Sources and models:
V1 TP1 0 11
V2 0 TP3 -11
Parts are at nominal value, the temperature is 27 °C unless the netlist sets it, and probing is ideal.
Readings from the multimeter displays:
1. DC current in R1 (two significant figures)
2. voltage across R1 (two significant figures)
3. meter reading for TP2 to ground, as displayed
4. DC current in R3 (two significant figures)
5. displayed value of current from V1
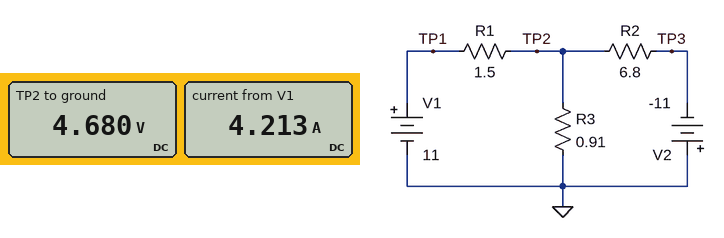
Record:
4.2 A
6.3 V
4.680 V
5.1 A
4.213 A
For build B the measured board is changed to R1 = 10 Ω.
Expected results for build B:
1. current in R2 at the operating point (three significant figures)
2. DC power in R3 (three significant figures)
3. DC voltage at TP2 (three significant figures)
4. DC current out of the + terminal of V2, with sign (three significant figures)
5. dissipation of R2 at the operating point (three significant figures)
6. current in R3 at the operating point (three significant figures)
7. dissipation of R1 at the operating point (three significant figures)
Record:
1.32 A
4.48 W
2.02 V
-1.32 A
11.9 W
2.22 A
8.07 W
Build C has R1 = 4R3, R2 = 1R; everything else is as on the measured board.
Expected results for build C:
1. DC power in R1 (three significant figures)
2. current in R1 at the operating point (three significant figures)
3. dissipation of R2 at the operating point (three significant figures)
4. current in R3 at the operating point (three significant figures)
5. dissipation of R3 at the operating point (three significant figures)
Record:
6.25 W
1.21 A
26.9 W
6.39 A
37.2 W
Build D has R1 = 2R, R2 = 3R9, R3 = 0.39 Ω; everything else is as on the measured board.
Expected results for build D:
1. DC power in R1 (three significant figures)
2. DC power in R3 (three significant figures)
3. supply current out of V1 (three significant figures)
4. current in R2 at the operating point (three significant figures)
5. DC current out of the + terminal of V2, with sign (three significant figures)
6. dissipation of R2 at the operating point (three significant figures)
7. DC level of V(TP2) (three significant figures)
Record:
36.1 W
16.1 W
4.25 A
2.18 A
-2.18 A
18.5 W
2.51 V
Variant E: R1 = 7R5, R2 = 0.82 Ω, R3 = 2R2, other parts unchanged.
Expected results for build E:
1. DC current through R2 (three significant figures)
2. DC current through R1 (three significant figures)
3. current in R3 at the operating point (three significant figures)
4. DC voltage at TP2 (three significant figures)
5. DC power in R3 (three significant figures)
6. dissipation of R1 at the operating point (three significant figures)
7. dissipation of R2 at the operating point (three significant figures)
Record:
3.37 A
369 mA
3.74 A
8.23 V
30.8 W
1.02 W
9.33 W
